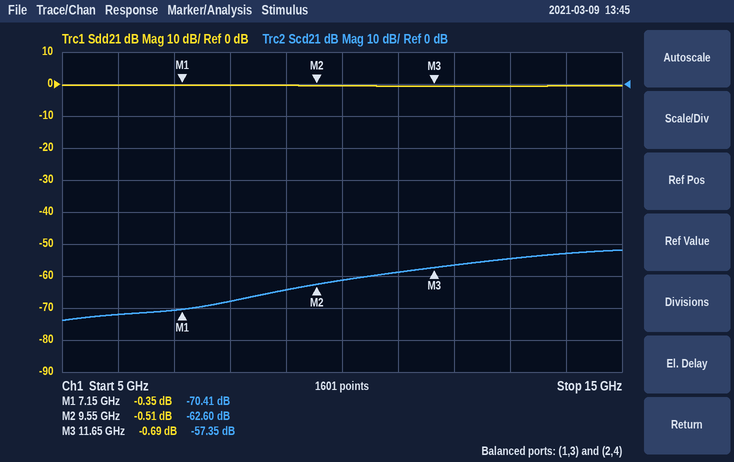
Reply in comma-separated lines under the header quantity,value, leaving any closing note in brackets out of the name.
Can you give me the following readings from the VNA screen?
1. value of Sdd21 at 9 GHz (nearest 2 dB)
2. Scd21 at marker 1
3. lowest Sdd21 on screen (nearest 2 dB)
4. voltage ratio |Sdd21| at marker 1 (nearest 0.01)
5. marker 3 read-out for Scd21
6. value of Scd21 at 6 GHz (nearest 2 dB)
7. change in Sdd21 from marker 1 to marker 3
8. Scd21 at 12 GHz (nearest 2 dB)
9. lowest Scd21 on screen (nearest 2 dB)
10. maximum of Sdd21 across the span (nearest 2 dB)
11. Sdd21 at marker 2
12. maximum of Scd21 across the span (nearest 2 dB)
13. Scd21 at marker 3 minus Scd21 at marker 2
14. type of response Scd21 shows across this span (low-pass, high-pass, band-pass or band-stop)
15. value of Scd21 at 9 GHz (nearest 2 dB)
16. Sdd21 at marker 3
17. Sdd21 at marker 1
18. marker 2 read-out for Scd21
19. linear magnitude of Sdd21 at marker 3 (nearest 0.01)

quantity,value
value of Sdd21 at 9 GHz,0 dB
Scd21 at marker 1,-70.41 dB
lowest Sdd21 on screen,0 dB
voltage ratio |Sdd21| at marker 1,0.96
marker 3 read-out for Scd21,-57.35 dB
value of Scd21 at 6 GHz,-72 dB
change in Sdd21 from marker 1 to marker 3,-0.34 dB
Scd21 at 12 GHz,-56 dB
lowest Scd21 on screen,-74 dB
maximum of Sdd21 across the span,0 dB
Sdd21 at marker 2,-0.51 dB
maximum of Scd21 across the span,-52 dB
Scd21 at marker 3 minus Scd21 at marker 2,5.25 dB
type of response Scd21 shows across this span,high-pass
value of Scd21 at 9 GHz,-64 dB
Sdd21 at marker 3,-0.69 dB
Sdd21 at marker 1,-0.35 dB
marker 2 read-out for Scd21,-62.60 dB
linear magnitude of Sdd21 at marker 3,0.92
